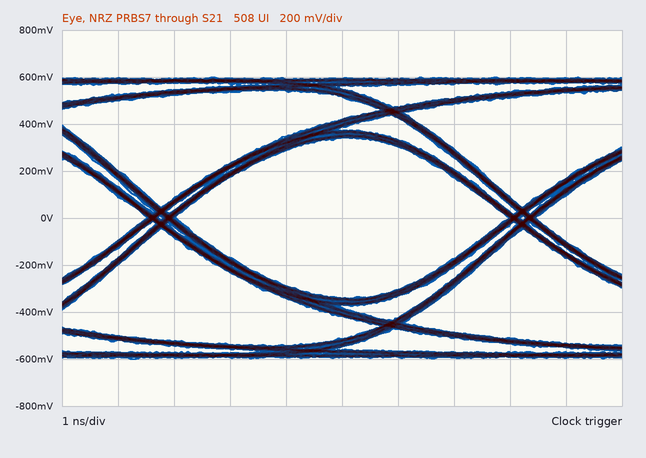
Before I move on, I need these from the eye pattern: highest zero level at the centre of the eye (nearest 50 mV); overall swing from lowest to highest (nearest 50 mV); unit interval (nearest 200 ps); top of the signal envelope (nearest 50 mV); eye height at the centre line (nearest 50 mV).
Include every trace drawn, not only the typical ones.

-350 mV
1.20 V
6.4 ns
600 mV
700 mV
